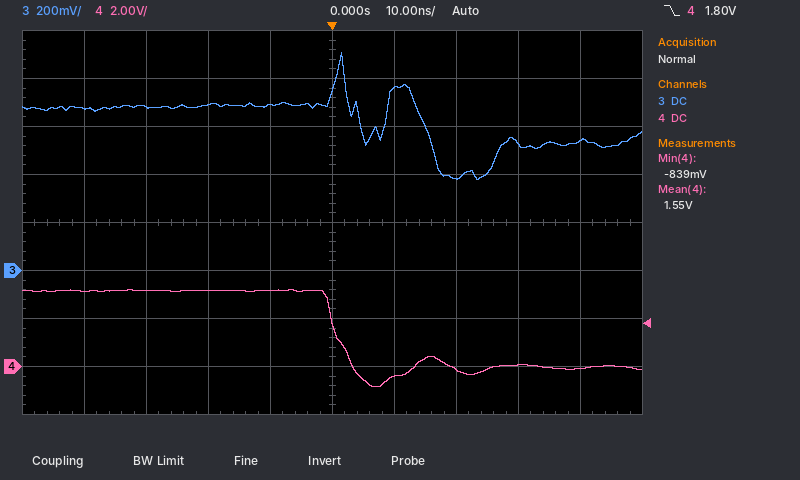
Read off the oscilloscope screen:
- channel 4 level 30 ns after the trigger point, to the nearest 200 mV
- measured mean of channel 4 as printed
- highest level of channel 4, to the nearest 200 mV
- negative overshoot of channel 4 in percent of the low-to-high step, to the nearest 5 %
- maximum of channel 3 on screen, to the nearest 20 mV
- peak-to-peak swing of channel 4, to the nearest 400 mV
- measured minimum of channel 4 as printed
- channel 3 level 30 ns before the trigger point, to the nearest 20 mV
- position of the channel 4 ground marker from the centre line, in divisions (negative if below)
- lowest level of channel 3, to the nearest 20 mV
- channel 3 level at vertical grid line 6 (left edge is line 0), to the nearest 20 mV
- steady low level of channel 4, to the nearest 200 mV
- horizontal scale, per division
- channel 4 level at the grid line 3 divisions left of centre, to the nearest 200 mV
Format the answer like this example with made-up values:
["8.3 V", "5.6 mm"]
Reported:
["0.0 V", "1.55 V", "3.2 V", "25 %", "900 mV", "4.0 V", "-839 mV", "680 mV", "-3.0 div", "380 mV", "760 mV", "0.0 V", "10 ns", "3.2 V"]
